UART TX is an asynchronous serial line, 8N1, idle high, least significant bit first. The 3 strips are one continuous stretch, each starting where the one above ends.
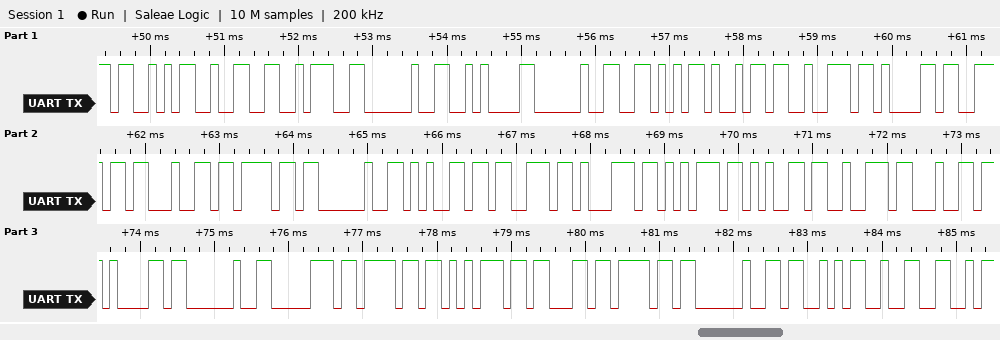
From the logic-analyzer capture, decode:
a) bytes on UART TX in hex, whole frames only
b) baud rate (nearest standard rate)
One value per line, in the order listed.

0x53 0x32 0x3A 0x20 0x0A 0x20 0x56 0x69 0x72 0x61 0x6E 0x64 0x6F 0x20 0x65 0x73 0x71 0x75 0x65 0x72 0x64 0x61 0x20 0x70 0x6F 0x75 0x63 0x6F 0x20 0x53 0x32
9600 baud
